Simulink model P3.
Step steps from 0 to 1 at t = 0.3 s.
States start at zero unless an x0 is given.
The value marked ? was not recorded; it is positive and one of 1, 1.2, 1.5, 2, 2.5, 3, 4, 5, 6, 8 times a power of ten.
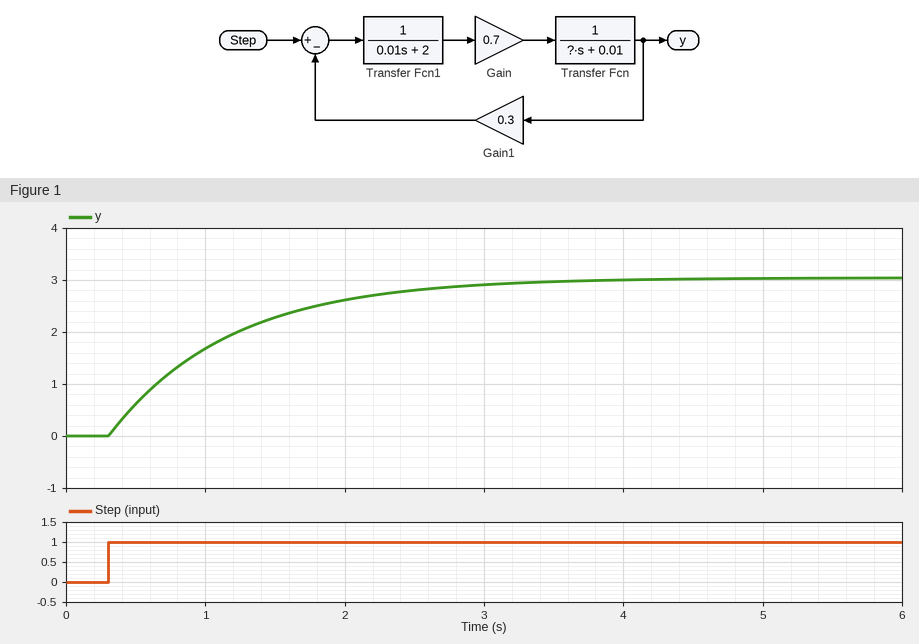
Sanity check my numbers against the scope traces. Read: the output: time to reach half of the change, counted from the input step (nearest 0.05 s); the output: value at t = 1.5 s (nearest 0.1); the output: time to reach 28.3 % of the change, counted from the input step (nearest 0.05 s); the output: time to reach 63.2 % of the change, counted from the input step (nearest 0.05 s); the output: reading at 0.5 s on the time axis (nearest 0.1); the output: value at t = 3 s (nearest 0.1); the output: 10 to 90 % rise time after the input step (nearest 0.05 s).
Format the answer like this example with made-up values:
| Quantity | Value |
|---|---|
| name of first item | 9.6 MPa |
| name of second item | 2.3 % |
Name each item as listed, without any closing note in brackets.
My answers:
| Quantity | Value |
|---|---|
| the output: time to reach half of the change, counted from the input step | 0.60 s |
| the output: value at t = 1.5 s | 2.3 |
| the output: time to reach 28.3 % of the change, counted from the input step | 0.30 s |
| the output: time to reach 63.2 % of the change, counted from the input step | 0.85 s |
| the output: reading at 0.5 s on the time axis | 0.6 |
| the output: value at t = 3 s | 2.9 |
| the output: 10 to 90 % rise time after the input step | 1.90 s |
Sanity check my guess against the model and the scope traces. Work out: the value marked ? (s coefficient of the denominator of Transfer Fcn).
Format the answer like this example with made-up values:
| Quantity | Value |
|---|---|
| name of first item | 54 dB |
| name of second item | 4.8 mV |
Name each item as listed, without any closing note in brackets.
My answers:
| Quantity | Value |
|---|---|
| the value marked ? | 0.1 |
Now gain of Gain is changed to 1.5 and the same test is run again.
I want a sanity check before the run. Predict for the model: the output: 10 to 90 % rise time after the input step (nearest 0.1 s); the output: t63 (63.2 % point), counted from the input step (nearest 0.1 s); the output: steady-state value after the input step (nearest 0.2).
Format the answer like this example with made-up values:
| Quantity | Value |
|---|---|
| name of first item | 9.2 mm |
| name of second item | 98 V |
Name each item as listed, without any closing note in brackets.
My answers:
| Quantity | Value |
|---|---|
| the output: 10 to 90 % rise time after the input step | 0.9 s |
| the output: t63 (63.2 % point), counted from the input step | 0.4 s |
| the output: steady-state value after the input step | 3.2 |
